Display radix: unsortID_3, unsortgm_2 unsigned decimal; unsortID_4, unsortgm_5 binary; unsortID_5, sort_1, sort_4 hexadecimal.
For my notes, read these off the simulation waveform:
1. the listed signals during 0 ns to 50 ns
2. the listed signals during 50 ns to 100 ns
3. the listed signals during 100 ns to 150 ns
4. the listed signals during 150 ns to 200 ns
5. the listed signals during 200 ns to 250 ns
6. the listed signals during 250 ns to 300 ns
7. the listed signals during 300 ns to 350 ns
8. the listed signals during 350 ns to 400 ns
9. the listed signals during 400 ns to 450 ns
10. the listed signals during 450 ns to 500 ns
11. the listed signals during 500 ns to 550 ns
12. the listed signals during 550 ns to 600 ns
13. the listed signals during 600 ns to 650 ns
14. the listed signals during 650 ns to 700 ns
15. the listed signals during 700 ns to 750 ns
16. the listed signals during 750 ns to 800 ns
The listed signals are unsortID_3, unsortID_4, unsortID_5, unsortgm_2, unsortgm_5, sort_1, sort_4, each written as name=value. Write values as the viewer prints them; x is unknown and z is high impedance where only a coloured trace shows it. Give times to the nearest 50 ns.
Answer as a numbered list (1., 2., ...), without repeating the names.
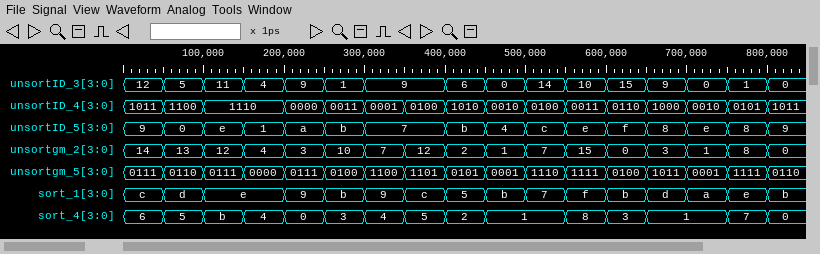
1. unsortID_3=12, unsortID_4=1011, unsortID_5=9, unsortgm_2=14, unsortgm_5=0111, sort_1=c, sort_4=6
2. unsortID_3=5, unsortID_4=1100, unsortID_5=0, unsortgm_2=13, unsortgm_5=0110, sort_1=d, sort_4=5
3. unsortID_3=11, unsortID_4=1110, unsortID_5=e, unsortgm_2=12, unsortgm_5=0111, sort_1=e, sort_4=b
4. unsortID_3=4, unsortID_4=1110, unsortID_5=1, unsortgm_2=4, unsortgm_5=0000, sort_1=e, sort_4=4
5. unsortID_3=9, unsortID_4=0000, unsortID_5=a, unsortgm_2=3, unsortgm_5=0111, sort_1=9, sort_4=0
6. unsortID_3=1, unsortID_4=0011, unsortID_5=b, unsortgm_2=10, unsortgm_5=0100, sort_1=b, sort_4=3
7. unsortID_3=9, unsortID_4=0001, unsortID_5=7, unsortgm_2=7, unsortgm_5=1100, sort_1=9, sort_4=4
8. unsortID_3=9, unsortID_4=0100, unsortID_5=7, unsortgm_2=12, unsortgm_5=1101, sort_1=c, sort_4=5
9. unsortID_3=6, unsortID_4=1010, unsortID_5=b, unsortgm_2=2, unsortgm_5=0101, sort_1=5, sort_4=2
10. unsortID_3=0, unsortID_4=0010, unsortID_5=4, unsortgm_2=1, unsortgm_5=0001, sort_1=b, sort_4=1
11. unsortID_3=14, unsortID_4=0100, unsortID_5=c, unsortgm_2=7, unsortgm_5=1110, sort_1=7, sort_4=1
12. unsortID_3=10, unsortID_4=0011, unsortID_5=e, unsortgm_2=15, unsortgm_5=1111, sort_1=f, sort_4=8
13. unsortID_3=15, unsortID_4=0110, unsortID_5=f, unsortgm_2=0, unsortgm_5=0100, sort_1=b, sort_4=3
14. unsortID_3=9, unsortID_4=1000, unsortID_5=8, unsortgm_2=3, unsortgm_5=1011, sort_1=d, sort_4=1
15. unsortID_3=0, unsortID_4=0010, unsortID_5=e, unsortgm_2=1, unsortgm_5=0001, sort_1=a, sort_4=1
16. unsortID_3=1, unsortID_4=0101, unsortID_5=8, unsortgm_2=8, unsortgm_5=1111, sort_1=e, sort_4=7
